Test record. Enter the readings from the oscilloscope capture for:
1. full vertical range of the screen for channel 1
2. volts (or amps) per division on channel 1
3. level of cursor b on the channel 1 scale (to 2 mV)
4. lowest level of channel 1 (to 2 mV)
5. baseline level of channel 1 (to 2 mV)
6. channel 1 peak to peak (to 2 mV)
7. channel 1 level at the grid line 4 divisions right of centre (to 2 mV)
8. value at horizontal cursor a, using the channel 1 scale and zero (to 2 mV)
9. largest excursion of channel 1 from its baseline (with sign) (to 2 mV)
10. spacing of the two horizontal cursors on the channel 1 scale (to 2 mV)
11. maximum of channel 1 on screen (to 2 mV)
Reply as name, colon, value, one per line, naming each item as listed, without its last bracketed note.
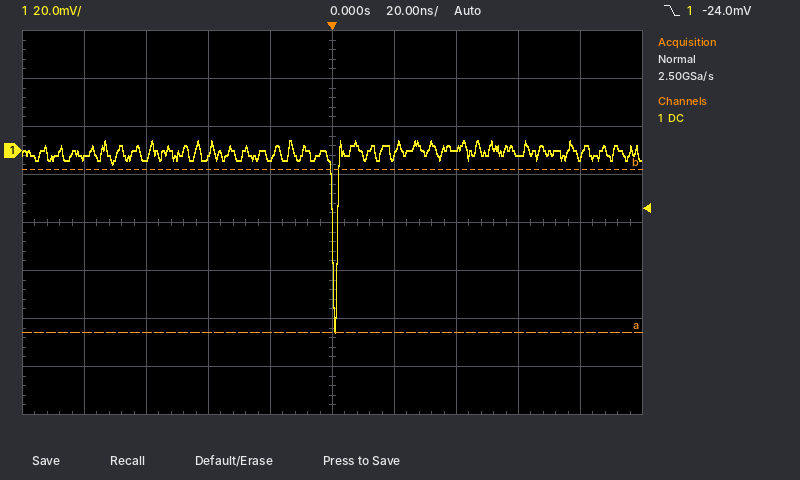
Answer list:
full vertical range of the screen for channel 1: 160 mV
volts (or amps) per division on channel 1: 20 mV
level of cursor b on the channel 1 scale: -8 mV
lowest level of channel 1: -76 mV
baseline level of channel 1: 0 mV
channel 1 peak to peak: 80 mV
channel 1 level at the grid line 4 divisions right of centre: -2 mV
value at horizontal cursor a, using the channel 1 scale and zero: -76 mV
largest excursion of channel 1 from its baseline (with sign): -76 mV
spacing of the two horizontal cursors on the channel 1 scale: 68 mV
maximum of channel 1 on screen: 4 mV
